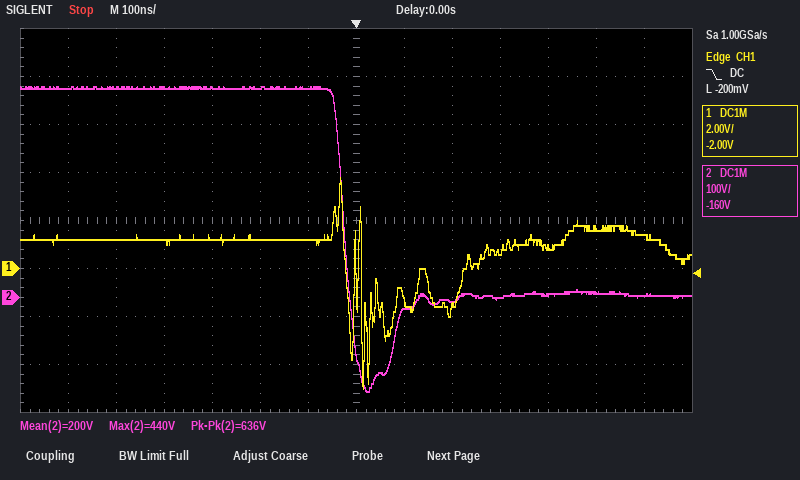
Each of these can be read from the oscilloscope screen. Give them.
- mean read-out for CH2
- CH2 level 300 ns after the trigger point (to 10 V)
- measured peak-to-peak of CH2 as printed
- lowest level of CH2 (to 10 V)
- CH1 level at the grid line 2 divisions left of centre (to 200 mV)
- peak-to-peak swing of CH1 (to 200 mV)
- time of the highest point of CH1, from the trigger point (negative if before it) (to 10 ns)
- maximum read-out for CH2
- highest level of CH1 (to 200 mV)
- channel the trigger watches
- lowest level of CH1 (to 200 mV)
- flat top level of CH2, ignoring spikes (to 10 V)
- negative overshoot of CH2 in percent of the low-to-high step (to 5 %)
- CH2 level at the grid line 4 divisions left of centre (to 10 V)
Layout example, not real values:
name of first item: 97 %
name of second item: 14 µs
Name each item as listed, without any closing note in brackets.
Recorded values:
mean read-out for CH2: 200 V
CH2 level 300 ns after the trigger point: 0 V
measured peak-to-peak of CH2 as printed: 636 V
lowest level of CH2: -200 V
CH1 level at the grid line 2 divisions left of centre: 1.2 V
peak-to-peak swing of CH1: 8.8 V
time of the highest point of CH1, from the trigger point (negative if before it): -30 ns
maximum read-out for CH2: 440 V
highest level of CH1: 3.8 V
channel the trigger watches: CH1
lowest level of CH1: -5.0 V
flat top level of CH2, ignoring spikes: 440 V
negative overshoot of CH2 in percent of the low-to-high step: 45 %
CH2 level at the grid line 4 divisions left of centre: 440 V
